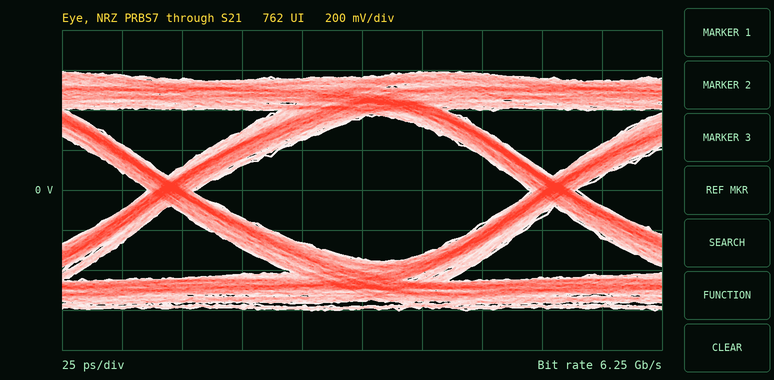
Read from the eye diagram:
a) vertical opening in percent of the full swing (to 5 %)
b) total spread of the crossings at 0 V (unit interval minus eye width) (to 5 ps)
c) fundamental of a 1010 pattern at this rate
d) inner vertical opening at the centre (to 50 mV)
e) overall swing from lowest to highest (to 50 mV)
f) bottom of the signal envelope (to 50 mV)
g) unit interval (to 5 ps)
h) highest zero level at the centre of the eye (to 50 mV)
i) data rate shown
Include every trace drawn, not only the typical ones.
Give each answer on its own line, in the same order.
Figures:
60 %
20 ps
3.125 GHz
700 mV
1.20 V
-600 mV
160 ps
-350 mV
6.25 Gb/s
